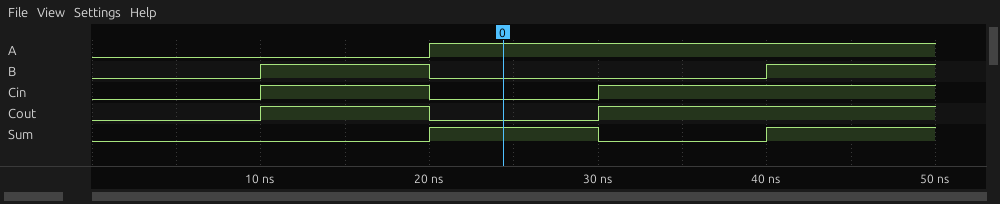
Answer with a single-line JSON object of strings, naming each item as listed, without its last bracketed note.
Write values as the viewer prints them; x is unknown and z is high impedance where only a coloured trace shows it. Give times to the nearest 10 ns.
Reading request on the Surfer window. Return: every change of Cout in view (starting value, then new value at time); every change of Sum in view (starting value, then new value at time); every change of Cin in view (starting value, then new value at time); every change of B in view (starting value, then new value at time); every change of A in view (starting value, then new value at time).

{"every change of Cout in view": "0, 1 at 10 ns, 0 at 20 ns, 1 at 30 ns", "every change of Sum in view": "0, 1 at 20 ns, 0 at 30 ns, 1 at 40 ns", "every change of Cin in view": "0, 1 at 10 ns, 0 at 20 ns, 1 at 30 ns", "every change of B in view": "0, 1 at 10 ns, 0 at 20 ns, 1 at 40 ns", "every change of A in view": "0, 1 at 20 ns"}
